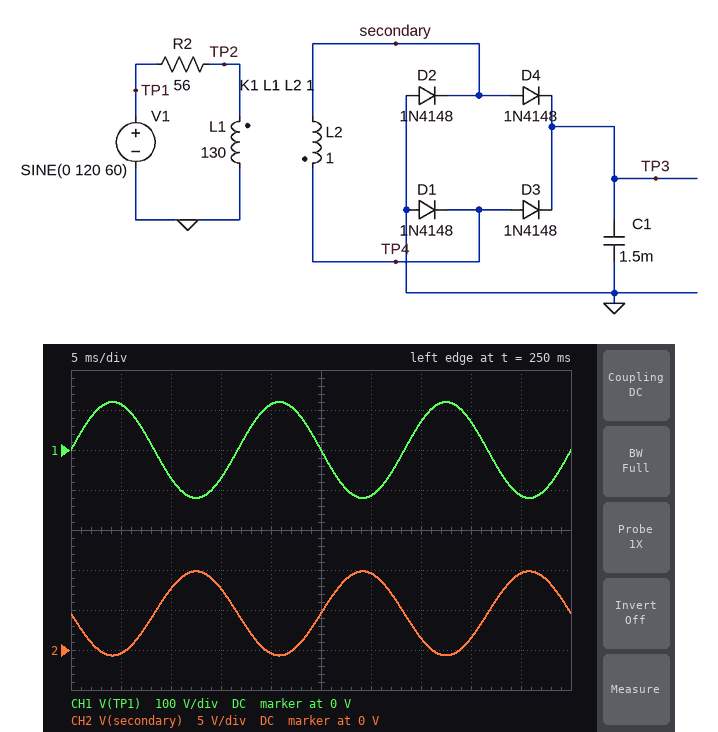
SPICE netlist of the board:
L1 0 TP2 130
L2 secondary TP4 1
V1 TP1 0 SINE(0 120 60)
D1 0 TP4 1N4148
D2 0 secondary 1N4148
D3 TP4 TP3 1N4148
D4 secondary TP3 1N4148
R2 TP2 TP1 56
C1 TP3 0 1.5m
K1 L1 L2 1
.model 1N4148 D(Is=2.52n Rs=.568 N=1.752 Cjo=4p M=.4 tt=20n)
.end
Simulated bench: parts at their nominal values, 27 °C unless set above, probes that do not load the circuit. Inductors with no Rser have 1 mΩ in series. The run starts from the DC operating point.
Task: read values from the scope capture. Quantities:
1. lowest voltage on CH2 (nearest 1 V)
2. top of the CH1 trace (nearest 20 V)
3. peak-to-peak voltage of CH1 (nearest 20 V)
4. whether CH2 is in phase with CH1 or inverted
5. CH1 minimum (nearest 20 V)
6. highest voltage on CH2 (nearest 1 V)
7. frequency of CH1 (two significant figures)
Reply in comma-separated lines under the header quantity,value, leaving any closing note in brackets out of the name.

quantity,value
lowest voltage on CH2,-1 V
top of the CH1 trace,120 V
peak-to-peak voltage of CH1,240 V
whether CH2 is in phase with CH1 or inverted,inverted
CH1 minimum,-120 V
highest voltage on CH2,10 V
frequency of CH1,60 Hz
